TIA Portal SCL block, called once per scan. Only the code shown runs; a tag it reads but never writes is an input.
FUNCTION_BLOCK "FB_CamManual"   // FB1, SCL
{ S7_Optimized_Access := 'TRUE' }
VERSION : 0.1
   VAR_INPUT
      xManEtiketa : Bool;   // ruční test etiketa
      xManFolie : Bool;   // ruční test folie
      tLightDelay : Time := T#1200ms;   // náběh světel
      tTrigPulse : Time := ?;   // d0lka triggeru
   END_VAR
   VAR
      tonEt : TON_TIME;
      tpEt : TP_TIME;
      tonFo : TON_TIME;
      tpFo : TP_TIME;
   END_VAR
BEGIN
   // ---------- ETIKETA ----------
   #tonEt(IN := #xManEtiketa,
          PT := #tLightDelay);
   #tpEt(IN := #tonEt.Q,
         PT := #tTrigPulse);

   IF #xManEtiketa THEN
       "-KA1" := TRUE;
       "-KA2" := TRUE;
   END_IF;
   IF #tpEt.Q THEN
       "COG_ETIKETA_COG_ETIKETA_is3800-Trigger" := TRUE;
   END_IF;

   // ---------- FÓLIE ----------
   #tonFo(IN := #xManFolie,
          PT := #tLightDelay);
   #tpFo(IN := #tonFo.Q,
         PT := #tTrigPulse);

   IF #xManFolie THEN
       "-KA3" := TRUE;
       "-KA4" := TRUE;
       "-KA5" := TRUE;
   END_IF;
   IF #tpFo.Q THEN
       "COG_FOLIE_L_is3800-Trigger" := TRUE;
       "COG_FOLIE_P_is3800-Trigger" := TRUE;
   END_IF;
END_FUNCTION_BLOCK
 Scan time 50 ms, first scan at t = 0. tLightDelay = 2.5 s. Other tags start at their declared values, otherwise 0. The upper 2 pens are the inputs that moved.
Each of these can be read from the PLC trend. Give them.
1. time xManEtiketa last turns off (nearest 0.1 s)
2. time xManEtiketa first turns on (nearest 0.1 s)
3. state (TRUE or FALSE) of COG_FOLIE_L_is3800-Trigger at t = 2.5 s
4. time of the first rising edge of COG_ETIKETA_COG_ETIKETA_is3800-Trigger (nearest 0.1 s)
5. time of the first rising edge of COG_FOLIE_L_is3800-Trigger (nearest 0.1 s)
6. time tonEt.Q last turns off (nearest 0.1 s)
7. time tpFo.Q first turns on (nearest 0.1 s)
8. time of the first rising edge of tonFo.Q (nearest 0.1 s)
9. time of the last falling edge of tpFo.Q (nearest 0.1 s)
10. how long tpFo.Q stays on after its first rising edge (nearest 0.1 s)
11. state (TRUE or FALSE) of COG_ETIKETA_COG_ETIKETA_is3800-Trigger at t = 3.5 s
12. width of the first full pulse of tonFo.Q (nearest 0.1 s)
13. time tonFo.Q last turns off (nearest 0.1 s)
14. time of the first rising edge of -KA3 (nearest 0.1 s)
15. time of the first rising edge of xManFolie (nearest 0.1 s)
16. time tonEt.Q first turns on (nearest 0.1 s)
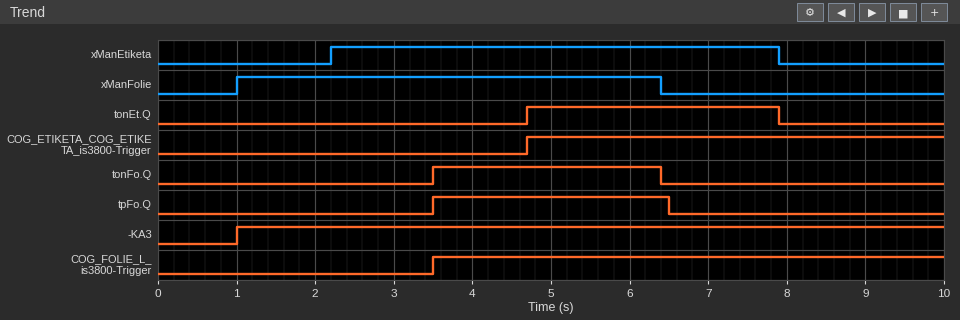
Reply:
7.9 s
2.2 s
FALSE
4.7 s
3.5 s
7.9 s
3.5 s
3.5 s
6.5 s
3.0 s
FALSE
2.9 s
6.4 s
1.0 s
1.0 s
4.7 s
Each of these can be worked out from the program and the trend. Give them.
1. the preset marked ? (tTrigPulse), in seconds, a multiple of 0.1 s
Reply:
3.0 s
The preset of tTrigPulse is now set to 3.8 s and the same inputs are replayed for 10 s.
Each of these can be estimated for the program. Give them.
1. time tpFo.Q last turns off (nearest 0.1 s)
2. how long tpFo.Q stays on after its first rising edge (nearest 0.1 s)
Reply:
7.3 s
3.8 s
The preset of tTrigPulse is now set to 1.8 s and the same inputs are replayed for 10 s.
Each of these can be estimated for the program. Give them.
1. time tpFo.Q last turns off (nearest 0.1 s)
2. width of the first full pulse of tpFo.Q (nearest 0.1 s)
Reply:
5.3 s
1.8 s
